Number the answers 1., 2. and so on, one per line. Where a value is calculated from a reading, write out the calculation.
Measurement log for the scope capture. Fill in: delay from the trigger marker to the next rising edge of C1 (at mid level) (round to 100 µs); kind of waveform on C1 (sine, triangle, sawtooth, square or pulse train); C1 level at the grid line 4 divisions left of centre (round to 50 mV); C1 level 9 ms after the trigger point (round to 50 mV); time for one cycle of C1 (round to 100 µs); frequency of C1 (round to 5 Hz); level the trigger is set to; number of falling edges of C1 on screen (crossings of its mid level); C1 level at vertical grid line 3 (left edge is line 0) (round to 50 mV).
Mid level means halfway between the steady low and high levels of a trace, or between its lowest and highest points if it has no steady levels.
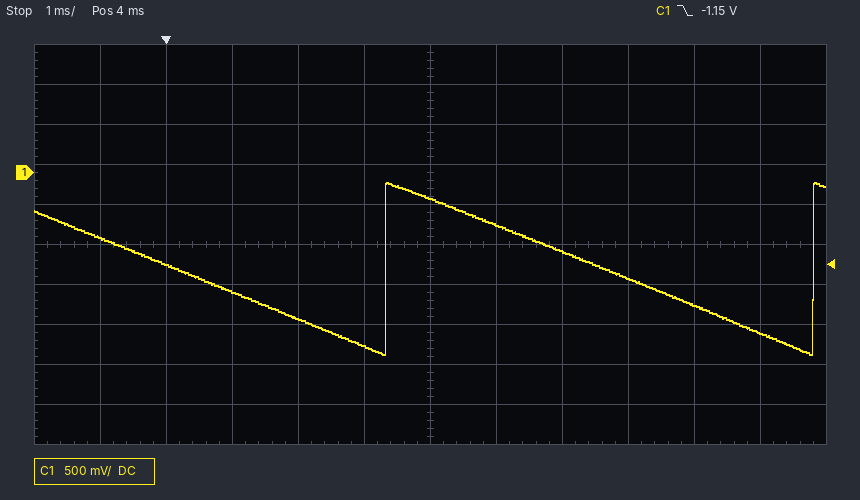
1. 3.3 ms
2. sawtooth
3. -1.15 V
4. -2.00 V
5. 6.5 ms
6. 1 / 6.5 ms ≈ 154 Hz, so 155 Hz to the nearest 5 Hz
7. -1.15 V
8. 2
9. -1.50 V
